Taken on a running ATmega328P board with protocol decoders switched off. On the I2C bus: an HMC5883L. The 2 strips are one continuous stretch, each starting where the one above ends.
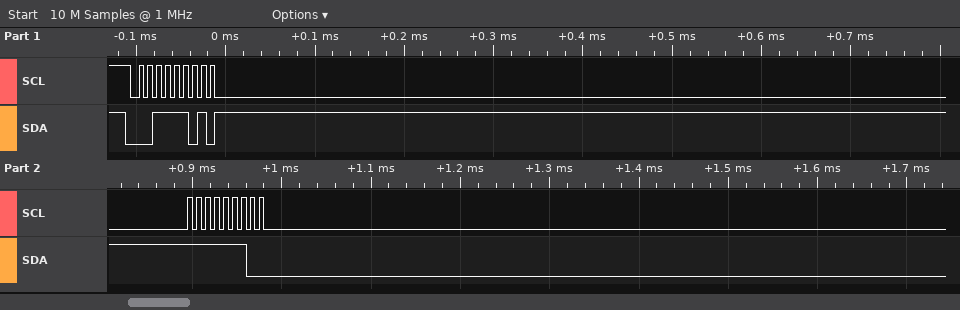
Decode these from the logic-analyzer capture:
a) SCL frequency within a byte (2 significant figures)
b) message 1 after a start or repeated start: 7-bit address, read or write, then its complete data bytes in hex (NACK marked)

100 kHz
0x1E read: FE
